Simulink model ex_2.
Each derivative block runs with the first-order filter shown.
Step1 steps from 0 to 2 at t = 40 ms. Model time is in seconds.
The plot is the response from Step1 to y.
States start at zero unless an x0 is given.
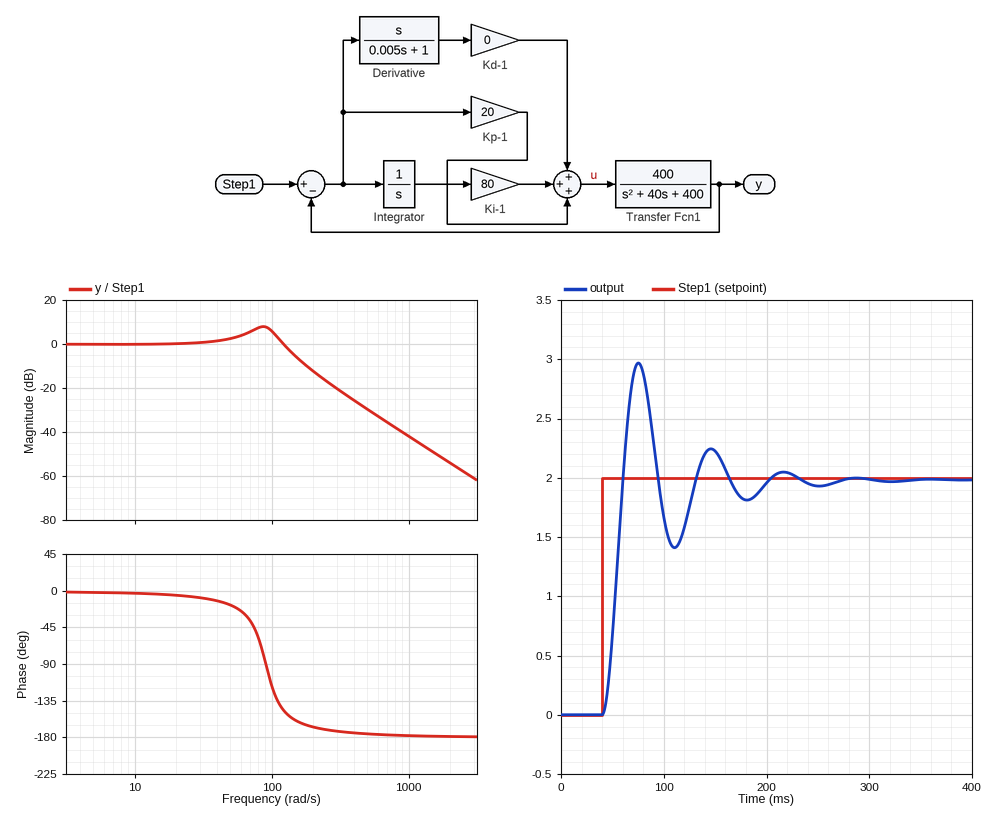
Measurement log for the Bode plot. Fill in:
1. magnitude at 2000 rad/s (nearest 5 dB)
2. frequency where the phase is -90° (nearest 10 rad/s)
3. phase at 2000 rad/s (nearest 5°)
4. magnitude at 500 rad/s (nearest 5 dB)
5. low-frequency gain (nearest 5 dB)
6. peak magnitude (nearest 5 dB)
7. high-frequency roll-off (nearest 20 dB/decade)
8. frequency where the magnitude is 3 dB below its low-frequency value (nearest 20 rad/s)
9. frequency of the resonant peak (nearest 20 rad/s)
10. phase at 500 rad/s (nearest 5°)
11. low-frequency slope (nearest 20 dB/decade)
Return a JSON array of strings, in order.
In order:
["-55 dB", "90 rad/s", "-180°", "-30 dB", "0 dB", "10 dB", "-40 dB/decade", "140 rad/s", "80 rad/s", "-175°", "0 dB/decade"]
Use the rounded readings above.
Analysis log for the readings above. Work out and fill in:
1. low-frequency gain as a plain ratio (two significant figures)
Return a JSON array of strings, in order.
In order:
["1.0"]
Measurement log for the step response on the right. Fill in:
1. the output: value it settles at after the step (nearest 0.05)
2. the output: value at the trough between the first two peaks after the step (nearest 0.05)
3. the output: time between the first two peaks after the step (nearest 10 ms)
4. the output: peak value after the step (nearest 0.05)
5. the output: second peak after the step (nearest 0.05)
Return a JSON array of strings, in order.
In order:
["2.00", "1.40", "70 ms", "2.95", "2.25"]
